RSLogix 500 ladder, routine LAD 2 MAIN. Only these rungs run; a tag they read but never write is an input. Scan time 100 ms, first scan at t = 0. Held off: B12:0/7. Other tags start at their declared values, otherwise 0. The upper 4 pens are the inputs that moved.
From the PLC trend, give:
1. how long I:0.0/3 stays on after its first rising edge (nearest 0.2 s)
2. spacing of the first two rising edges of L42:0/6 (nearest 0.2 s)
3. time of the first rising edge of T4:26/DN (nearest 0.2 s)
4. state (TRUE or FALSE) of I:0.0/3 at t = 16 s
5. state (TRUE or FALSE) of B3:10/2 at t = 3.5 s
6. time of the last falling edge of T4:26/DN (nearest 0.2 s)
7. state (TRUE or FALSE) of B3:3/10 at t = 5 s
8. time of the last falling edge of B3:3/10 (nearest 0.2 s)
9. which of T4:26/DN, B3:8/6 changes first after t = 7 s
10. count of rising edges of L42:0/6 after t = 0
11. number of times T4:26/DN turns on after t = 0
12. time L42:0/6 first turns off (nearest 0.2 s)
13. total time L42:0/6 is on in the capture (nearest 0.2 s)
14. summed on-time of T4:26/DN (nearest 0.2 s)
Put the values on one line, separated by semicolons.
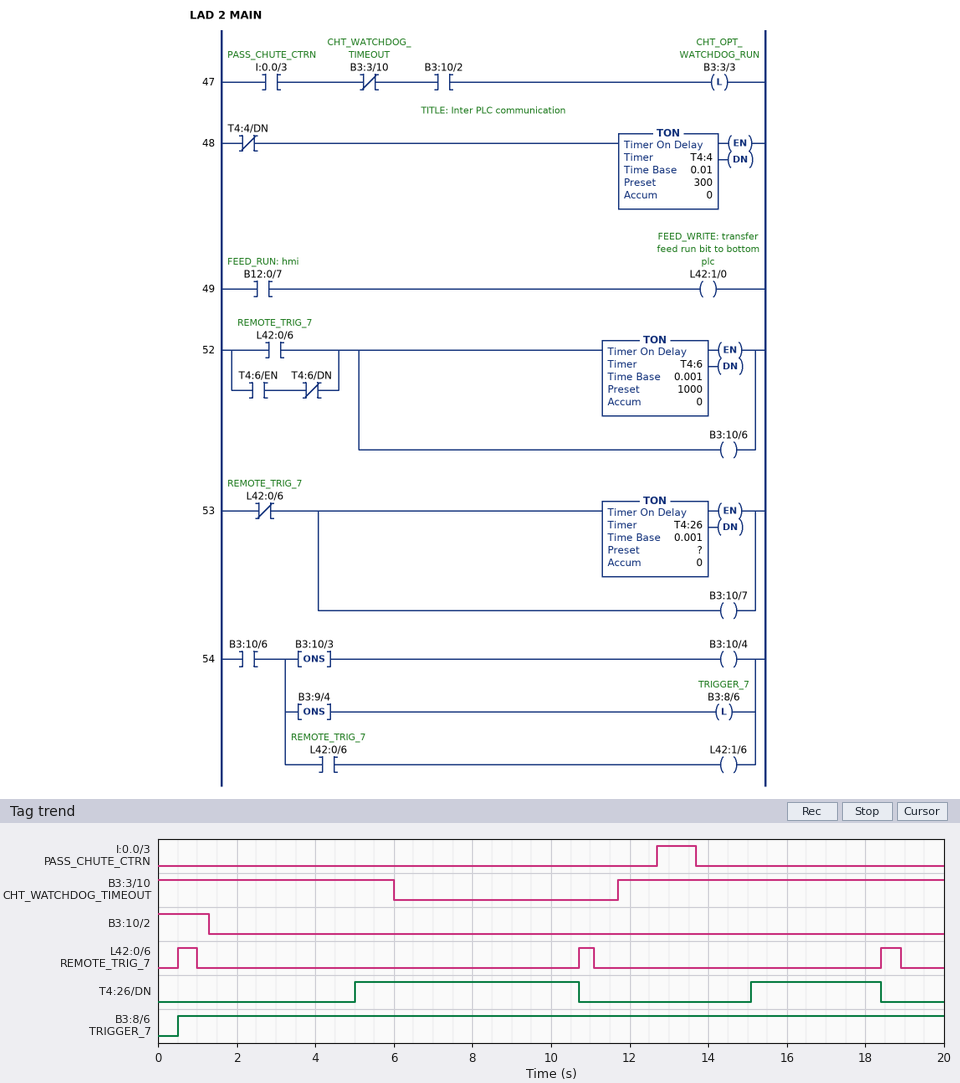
1.0 s; 10.2 s; 5.0 s; FALSE; FALSE; 18.4 s; TRUE; 6.0 s; T4:26/DN; 3; 2; 1.0 s; 1.4 s; 9.0 s
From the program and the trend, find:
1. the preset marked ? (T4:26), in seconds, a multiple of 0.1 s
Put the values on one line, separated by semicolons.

4.0 s
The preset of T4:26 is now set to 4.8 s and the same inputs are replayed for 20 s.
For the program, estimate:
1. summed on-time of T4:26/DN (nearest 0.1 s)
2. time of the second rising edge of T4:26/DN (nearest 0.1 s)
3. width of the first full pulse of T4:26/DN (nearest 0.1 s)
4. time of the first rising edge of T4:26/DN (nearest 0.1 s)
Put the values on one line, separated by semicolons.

7.4 s; 15.9 s; 4.9 s; 5.8 s
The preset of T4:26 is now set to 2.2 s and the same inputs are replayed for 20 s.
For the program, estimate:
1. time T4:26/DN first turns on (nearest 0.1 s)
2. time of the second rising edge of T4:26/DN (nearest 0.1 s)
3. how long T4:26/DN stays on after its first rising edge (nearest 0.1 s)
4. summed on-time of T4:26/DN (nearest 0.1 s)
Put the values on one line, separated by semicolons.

3.2 s; 13.3 s; 7.5 s; 12.6 s
